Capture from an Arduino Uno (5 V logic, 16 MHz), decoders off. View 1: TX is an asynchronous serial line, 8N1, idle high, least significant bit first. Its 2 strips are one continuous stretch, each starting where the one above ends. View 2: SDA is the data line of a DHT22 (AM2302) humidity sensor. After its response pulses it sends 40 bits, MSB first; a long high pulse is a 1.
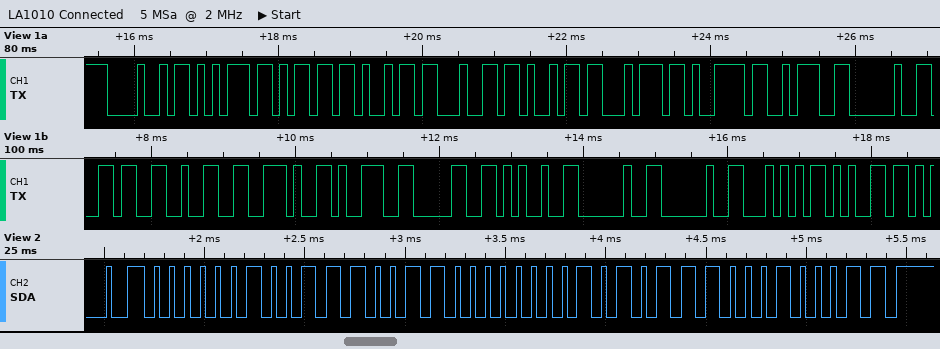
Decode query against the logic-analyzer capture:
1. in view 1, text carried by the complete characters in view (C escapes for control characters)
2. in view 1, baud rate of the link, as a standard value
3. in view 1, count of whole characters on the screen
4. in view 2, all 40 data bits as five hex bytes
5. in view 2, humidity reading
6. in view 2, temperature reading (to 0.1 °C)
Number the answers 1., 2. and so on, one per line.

1. "Humidity: 62.90%  Te"
2. 9600 baud
3. 20
4. 02 73 00 AE 23
5. 62.7 %
6. 17.4 °C
